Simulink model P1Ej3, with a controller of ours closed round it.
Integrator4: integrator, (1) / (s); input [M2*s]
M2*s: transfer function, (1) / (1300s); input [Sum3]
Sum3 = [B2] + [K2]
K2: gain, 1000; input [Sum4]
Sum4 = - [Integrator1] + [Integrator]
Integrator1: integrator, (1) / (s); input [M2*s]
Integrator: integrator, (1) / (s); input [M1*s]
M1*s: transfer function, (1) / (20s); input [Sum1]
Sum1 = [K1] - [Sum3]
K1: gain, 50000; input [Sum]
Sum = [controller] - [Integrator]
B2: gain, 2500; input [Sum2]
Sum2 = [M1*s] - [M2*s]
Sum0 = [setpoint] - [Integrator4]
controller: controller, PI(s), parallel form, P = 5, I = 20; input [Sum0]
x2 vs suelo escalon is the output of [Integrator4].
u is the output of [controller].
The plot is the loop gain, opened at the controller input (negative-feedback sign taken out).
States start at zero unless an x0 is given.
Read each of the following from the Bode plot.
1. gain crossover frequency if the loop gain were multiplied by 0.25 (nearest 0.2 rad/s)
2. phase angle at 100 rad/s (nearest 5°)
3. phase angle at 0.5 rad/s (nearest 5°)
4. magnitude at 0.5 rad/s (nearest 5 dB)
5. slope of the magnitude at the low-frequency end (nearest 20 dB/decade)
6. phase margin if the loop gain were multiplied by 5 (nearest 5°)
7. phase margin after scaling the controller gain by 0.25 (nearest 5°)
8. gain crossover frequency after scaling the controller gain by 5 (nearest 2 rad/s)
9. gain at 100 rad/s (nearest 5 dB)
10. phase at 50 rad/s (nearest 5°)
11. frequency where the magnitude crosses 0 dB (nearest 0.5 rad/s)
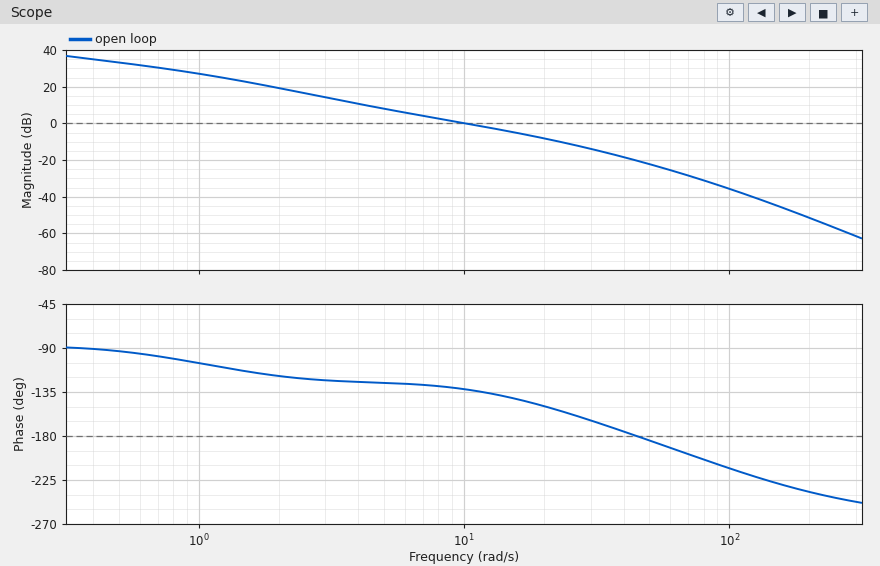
3.6 rad/s
-215°
-95°
35 dB
-20 dB/decade
15°
55°
30 rad/s
-35 dB
-185°
10.0 rad/s
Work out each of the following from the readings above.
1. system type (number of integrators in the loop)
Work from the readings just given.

1
